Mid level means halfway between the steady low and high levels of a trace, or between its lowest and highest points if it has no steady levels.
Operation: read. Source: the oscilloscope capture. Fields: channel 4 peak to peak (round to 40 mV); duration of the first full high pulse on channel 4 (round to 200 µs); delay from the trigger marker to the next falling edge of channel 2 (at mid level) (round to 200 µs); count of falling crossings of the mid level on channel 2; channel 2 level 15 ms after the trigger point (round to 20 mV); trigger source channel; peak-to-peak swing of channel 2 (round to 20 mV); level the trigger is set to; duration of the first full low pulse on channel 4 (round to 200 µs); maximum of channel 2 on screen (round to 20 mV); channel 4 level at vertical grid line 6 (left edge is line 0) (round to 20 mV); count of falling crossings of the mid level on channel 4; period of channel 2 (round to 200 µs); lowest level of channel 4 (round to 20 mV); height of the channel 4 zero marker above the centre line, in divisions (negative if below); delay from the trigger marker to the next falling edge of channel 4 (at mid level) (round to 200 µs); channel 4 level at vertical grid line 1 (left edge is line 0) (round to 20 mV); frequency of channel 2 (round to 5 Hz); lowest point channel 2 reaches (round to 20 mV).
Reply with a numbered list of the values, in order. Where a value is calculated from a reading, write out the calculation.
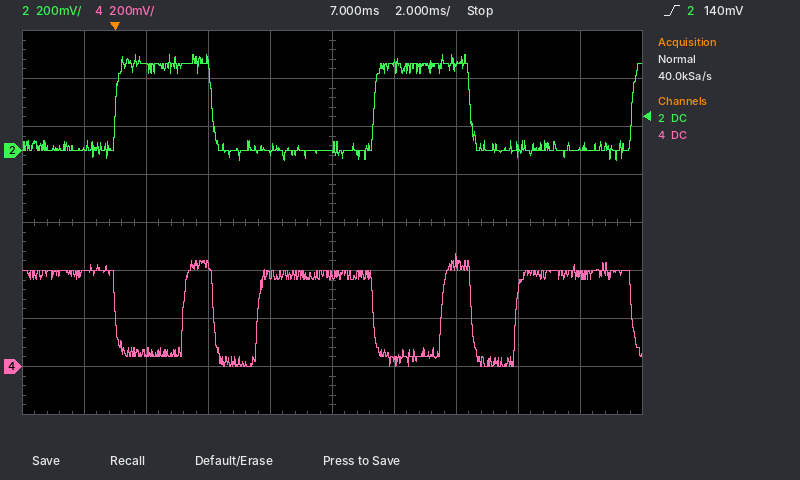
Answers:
1. 480 mV
2. 1.0 ms
3. 3.2 ms
4. 2
5. 0 mV
6. channel 2
7. 400 mV − (-40 mV) = 440 mV
8. 140 mV
9. 2.2 ms
10. 400 mV
11. 20 mV
12. 5
13. 8.4 ms
14. 0 mV
15. -3.0 div
16. 3.2 ms
17. 400 mV
18. 1 / 8.4 ms ≈ 119 Hz, so 120 Hz to the nearest 5 Hz
19. -40 mV
